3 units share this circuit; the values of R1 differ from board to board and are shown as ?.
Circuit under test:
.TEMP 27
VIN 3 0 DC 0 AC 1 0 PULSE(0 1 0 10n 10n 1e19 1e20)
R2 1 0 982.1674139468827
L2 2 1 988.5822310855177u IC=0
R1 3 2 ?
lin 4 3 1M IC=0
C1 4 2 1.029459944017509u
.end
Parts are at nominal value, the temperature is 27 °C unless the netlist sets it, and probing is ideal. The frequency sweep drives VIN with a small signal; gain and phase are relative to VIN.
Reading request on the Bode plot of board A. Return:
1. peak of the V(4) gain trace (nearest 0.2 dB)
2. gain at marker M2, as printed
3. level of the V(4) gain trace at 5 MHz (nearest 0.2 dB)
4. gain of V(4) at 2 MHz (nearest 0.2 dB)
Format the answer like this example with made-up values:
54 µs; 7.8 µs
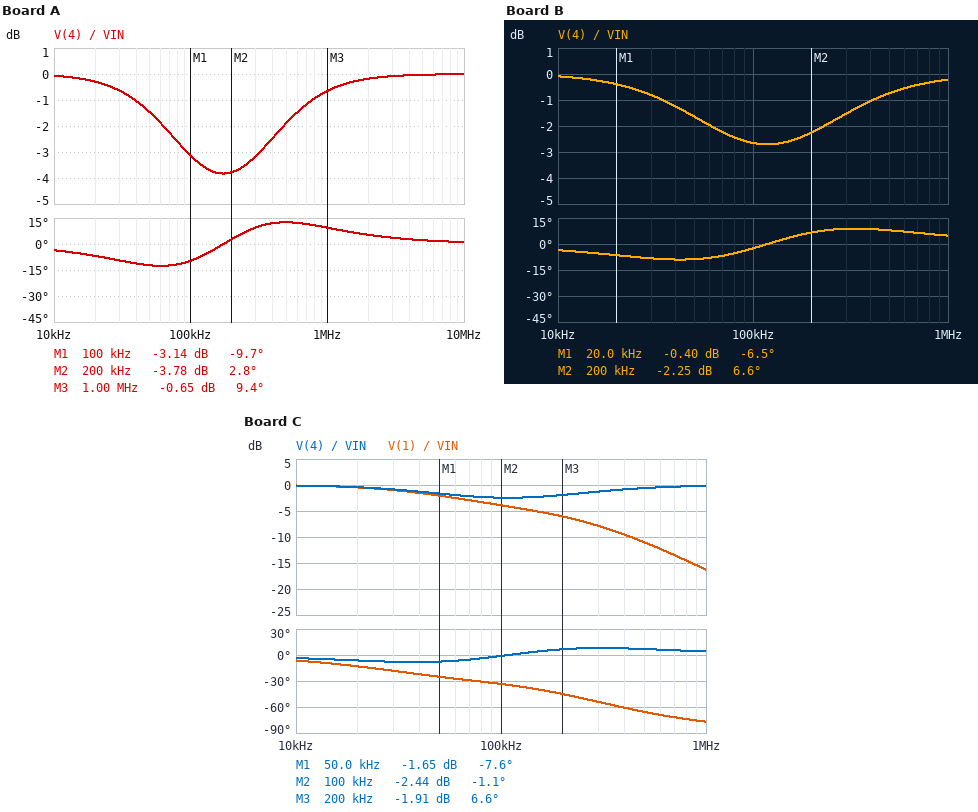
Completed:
0 dB; -3.78 dB; 0 dB; -0.2 dB
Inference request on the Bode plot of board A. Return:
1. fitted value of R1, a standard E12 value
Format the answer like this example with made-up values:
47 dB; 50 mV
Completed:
1.2 kΩ
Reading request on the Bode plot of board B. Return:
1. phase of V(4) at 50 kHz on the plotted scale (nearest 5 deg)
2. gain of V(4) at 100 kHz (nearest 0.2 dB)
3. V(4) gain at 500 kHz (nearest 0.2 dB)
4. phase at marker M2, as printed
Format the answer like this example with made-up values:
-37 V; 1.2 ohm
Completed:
-10 deg; -2.6 dB; -0.8 dB; 6.6 deg
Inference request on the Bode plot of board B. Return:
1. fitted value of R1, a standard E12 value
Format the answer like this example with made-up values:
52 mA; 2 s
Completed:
560 Ω
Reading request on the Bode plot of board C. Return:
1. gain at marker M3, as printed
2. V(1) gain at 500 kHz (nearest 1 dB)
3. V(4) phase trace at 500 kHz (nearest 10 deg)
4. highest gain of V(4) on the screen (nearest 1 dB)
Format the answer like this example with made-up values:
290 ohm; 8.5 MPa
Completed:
-1.91 dB; -11 dB; 10 deg; 0 dB
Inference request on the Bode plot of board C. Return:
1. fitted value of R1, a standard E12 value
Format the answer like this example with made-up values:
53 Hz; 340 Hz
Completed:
470 Ω
